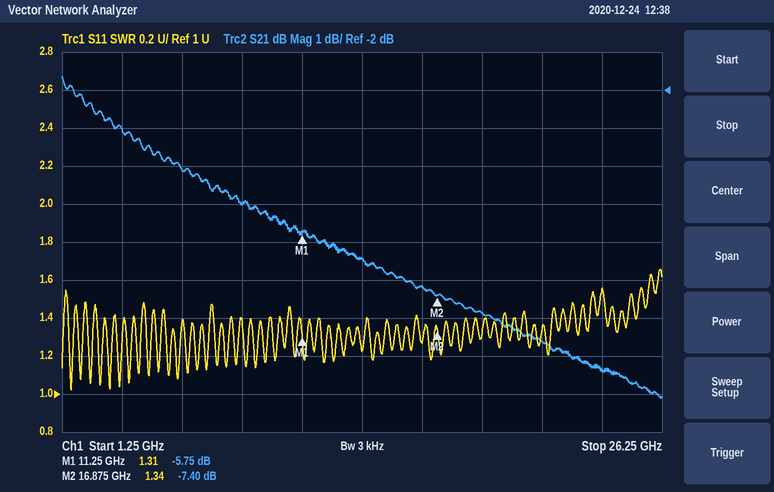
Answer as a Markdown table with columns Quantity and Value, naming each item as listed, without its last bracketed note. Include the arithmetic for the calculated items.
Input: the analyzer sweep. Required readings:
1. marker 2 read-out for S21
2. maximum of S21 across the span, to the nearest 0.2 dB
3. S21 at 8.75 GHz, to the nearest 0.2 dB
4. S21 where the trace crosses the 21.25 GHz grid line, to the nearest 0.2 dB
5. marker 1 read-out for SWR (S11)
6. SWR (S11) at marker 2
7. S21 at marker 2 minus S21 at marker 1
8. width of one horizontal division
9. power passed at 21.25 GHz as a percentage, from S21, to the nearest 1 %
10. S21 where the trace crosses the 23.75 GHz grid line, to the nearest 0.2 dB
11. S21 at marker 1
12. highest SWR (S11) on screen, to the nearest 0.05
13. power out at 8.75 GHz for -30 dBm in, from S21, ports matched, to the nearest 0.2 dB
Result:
| Quantity | Value |
|---|---|
| marker 2 read-out for S21 | -7.40 dB |
| maximum of S21 across the span, to the nearest 0.2 dB | -1.6 dB |
| S21 at 8.75 GHz, to the nearest 0.2 dB | -5.0 dB |
| S21 where the trace crosses the 21.25 GHz grid line, to the nearest 0.2 dB | -8.6 dB |
| marker 1 read-out for SWR | 1.31 |
| SWR (S11) at marker 2 | 1.34 |
| S21 at marker 2 minus S21 at marker 1 | -7.4 − (-5.75) = -1.65 dB |
| width of one horizontal division | 2.5 GHz |
| power passed at 21.25 GHz as a percentage, from S21, to the nearest 1 % | 10^(-8.6/10) ≈ 14 % |
| S21 where the trace crosses the 23.75 GHz grid line, to the nearest 0.2 dB | -9.4 dB |
| S21 at marker 1 | -5.75 dB |
| highest SWR (S11) on screen, to the nearest 0.05 | 1.65 |
| power out at 8.75 GHz for -30 dBm in, from S21, ports matched, to the nearest 0.2 dB | -30 dBm + (-5.0 dB) = -35.0 dBm |
